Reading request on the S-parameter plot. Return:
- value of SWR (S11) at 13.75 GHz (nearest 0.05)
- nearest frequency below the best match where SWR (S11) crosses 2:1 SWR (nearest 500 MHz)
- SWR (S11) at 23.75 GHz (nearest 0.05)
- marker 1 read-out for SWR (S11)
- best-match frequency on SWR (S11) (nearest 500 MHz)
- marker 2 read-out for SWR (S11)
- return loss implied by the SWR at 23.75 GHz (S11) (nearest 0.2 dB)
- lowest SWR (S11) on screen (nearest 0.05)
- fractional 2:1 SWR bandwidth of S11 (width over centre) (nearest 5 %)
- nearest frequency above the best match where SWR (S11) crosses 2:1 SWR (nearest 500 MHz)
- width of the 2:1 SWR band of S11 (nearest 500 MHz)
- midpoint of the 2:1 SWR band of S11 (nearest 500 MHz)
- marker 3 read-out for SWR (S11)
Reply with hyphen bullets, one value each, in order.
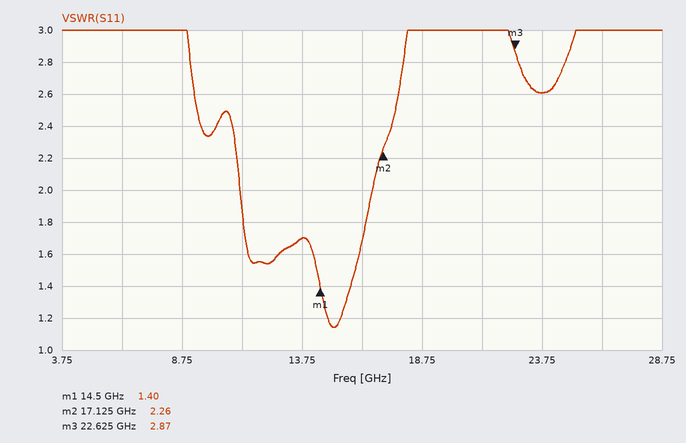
- 1.70
- 11.0 GHz
- 2.60
- 1.40
- 15.0 GHz
- 2.26
- 7.0 dB
- 1.15
- 40 %
- 16.5 GHz
- 5.5 GHz
- 14.0 GHz
- 2.87
